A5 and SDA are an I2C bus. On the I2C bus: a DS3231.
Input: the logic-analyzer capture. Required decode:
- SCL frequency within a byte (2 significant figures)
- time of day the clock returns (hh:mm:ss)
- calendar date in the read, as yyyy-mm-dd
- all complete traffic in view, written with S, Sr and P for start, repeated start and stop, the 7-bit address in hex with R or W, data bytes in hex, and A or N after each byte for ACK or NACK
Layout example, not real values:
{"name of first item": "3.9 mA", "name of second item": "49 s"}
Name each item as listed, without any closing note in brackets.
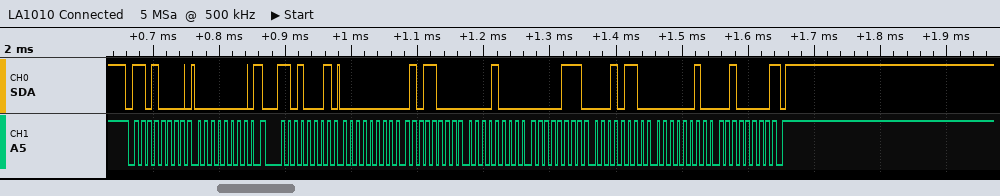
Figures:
{"SCL frequency within a byte": "100 kHz", "time of day the clock returns": "08:58:00", "calendar date in the read, as yyyy-mm-dd": "2020-02-16", "all complete traffic in view, written with S, Sr and P for start, repeated start and stop, the 7-bit address in hex with R or W, data bytes in hex, and A or N after each byte for ACK or NACK": "S 68W A 00 A Sr 68R A 00 A 58 A 08 A 07 A 16 A 02 A 20 N P"}
